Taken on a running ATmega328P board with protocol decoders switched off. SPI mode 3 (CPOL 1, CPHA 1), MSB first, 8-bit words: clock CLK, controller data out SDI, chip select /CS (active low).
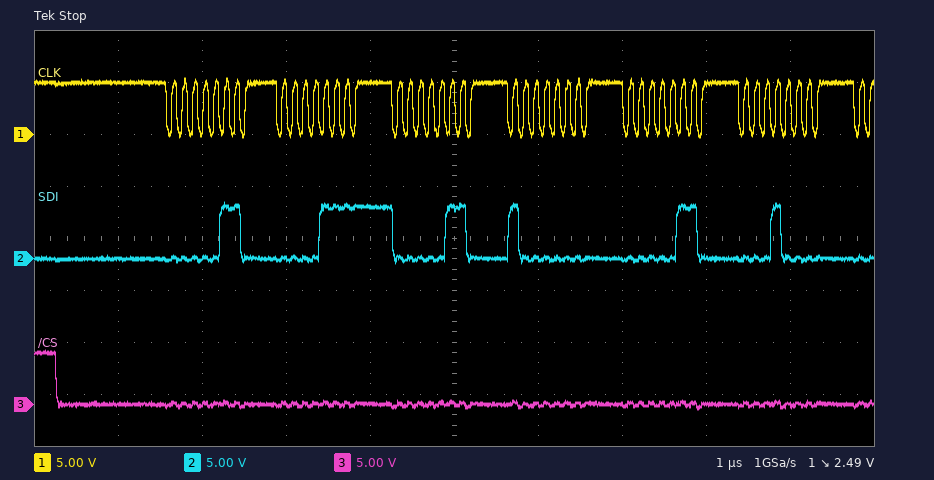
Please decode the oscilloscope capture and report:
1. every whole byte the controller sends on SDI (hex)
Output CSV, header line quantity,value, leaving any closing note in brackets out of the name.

quantity,value
every whole byte the controller sends on SDI,06 0F 06 80 06 10
